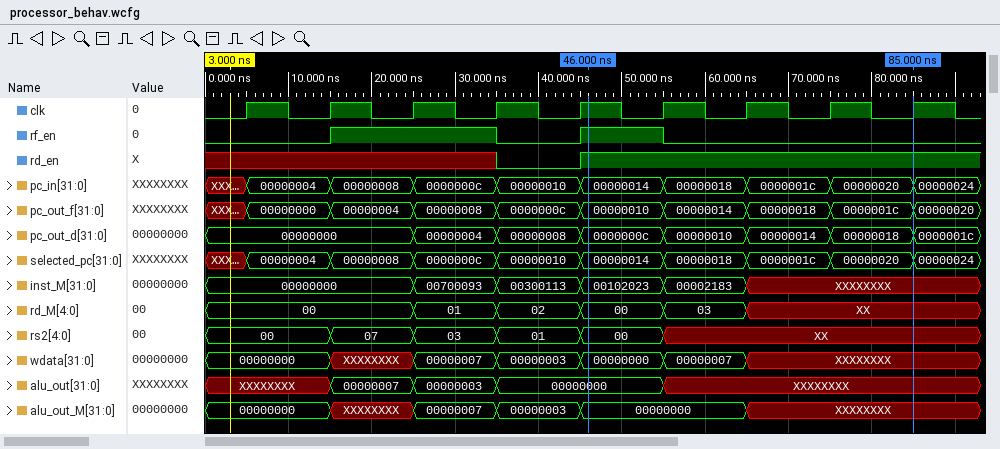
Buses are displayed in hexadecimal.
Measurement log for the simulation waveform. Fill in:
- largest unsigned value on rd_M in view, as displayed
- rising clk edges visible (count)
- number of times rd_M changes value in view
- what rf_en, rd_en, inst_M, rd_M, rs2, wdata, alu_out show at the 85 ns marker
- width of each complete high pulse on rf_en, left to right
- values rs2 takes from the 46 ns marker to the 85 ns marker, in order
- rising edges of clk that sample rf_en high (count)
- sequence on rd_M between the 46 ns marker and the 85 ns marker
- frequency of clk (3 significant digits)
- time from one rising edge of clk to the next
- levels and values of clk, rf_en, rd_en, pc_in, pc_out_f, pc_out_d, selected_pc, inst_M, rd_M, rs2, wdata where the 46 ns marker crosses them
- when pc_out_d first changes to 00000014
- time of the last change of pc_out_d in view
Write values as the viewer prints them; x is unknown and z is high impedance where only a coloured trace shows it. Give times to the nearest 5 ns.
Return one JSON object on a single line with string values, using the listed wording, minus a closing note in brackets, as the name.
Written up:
{"largest unsigned value on rd_M in view, as displayed": "03", "rising clk edges visible": "9", "number of times rd_M changes value in view": "5", "what rf_en, rd_en, inst_M, rd_M, rs2, wdata, alu_out show at the 85 ns marker": "rf_en=0, rd_en=1, inst_M=XXXXXXXX, rd_M=XX, rs2=XX, wdata=XXXXXXXX, alu_out=XXXXXXXX", "width of each complete high pulse on rf_en, left to right": "20 ns, 10 ns", "values rs2 takes from the 46 ns marker to the 85 ns marker, in order": "00, XX", "rising edges of clk that sample rf_en high": "3", "sequence on rd_M between the 46 ns marker and the 85 ns marker": "00, 03, XX", "frequency of clk": "100 MHz", "time from one rising edge of clk to the next": "10 ns", "levels and values of clk, rf_en, rd_en, pc_in, pc_out_f, pc_out_d, selected_pc, inst_M, rd_M, rs2, wdata where the 46 ns marker crosses them": "clk=1, rf_en=1, rd_en=1, pc_in=00000014, pc_out_f=00000010, pc_out_d=0000000c, selected_pc=00000014, inst_M=00102023, rd_M=00, rs2=00, wdata=00000000", "when pc_out_d first changes to 00000014": "65 ns", "time of the last change of pc_out_d in view": "85 ns"}
